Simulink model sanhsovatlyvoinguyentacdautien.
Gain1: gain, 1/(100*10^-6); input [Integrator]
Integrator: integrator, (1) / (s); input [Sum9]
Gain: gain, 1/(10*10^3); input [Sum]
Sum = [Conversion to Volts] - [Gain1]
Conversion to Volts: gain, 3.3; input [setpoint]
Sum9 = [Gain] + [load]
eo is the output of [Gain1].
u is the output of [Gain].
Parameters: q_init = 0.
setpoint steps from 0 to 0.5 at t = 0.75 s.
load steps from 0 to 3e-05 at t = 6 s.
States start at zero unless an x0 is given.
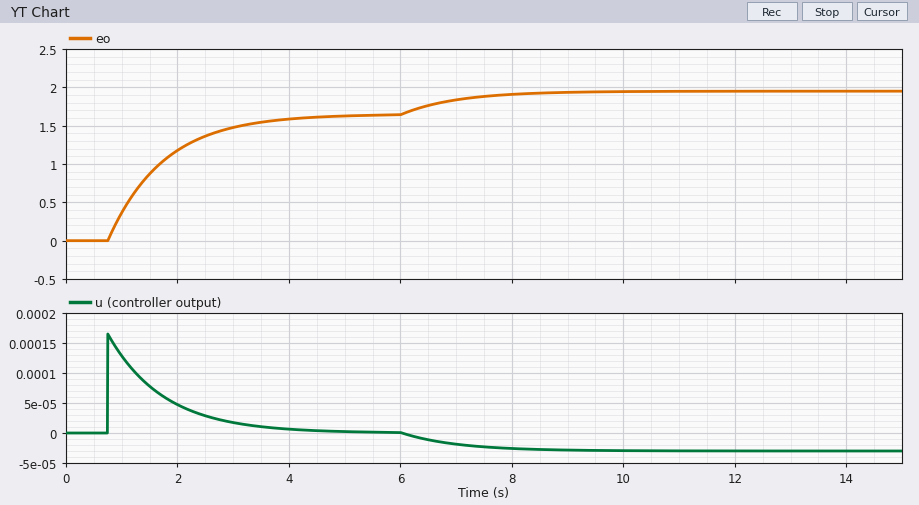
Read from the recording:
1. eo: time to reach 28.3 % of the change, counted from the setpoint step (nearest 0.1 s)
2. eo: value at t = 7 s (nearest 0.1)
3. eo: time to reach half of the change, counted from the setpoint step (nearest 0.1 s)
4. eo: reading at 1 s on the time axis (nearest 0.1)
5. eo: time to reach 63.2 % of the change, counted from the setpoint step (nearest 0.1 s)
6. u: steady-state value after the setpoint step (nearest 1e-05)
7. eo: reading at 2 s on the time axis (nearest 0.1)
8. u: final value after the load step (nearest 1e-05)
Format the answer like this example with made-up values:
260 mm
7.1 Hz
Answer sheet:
0.3 s
1.8
0.7 s
0.4
1.0 s
0.00000
1.2
-0.00003
